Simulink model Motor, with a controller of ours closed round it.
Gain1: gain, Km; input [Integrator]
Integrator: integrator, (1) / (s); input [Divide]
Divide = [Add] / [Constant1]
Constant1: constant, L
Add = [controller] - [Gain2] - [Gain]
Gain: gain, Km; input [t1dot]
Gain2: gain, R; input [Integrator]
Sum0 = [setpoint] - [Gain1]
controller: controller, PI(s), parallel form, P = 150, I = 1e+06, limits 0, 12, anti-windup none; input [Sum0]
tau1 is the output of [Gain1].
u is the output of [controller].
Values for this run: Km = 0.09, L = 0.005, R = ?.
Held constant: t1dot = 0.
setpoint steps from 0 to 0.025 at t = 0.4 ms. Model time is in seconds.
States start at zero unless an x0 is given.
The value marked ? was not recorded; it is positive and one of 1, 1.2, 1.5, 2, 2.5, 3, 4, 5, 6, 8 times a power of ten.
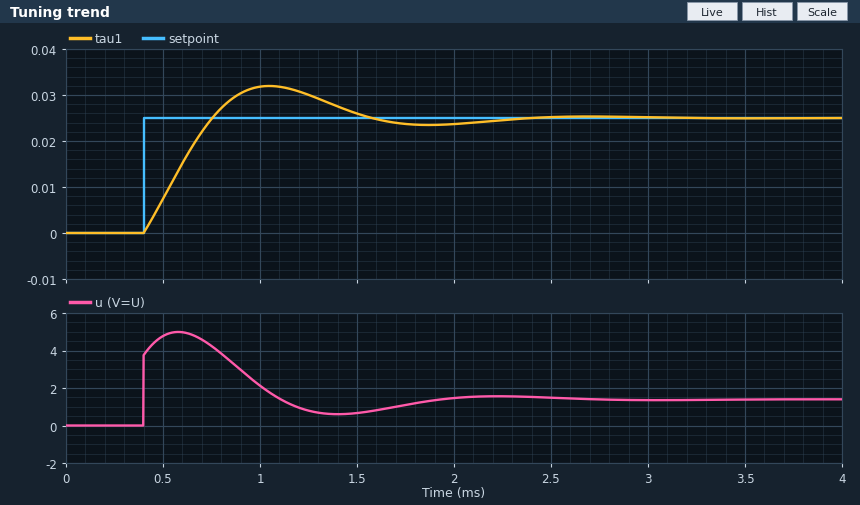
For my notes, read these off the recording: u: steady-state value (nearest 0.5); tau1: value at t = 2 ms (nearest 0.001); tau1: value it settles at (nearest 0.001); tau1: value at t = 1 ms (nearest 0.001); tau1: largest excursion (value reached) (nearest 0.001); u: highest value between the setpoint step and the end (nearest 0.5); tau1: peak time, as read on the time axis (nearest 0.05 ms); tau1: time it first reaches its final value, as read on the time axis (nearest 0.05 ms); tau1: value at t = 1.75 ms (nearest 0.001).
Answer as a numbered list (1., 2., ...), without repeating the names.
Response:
1. 1.5
2. 0.024
3. 0.025
4. 0.032
5. 0.032
6. 5.0
7. 1.05 ms
8. 0.75 ms
9. 0.024
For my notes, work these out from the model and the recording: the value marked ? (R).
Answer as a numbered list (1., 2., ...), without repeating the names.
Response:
1. 5
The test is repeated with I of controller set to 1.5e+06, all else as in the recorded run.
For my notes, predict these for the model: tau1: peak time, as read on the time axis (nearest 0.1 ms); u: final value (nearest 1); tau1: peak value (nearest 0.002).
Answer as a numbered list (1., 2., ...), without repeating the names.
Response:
1. 0.9 ms
2. 1
3. 0.034
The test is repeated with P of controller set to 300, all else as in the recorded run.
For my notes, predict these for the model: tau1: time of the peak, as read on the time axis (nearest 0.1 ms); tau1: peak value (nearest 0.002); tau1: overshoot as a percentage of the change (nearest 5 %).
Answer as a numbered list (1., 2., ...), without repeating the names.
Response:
1. 1.0 ms
2. 0.028
3. 15 %
